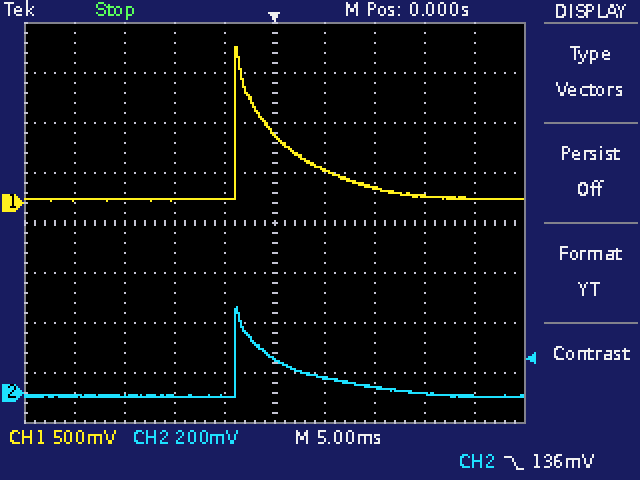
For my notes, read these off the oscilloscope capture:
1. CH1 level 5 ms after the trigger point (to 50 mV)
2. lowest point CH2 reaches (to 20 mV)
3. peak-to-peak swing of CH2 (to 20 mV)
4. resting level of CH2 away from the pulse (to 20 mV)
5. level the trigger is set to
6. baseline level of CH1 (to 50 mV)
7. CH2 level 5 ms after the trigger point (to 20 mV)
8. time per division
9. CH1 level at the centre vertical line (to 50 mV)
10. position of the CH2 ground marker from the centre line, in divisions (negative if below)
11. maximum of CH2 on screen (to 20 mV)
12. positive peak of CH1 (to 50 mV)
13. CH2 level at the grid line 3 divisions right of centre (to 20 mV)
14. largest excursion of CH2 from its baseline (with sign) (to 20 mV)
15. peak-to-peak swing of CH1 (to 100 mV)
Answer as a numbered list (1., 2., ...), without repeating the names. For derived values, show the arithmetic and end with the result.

1. 350 mV
2. -20 mV
3. 340 mV − (-20 mV) = 360 mV
4. -20 mV
5. 136 mV
6. 50 mV
7. 60 mV
8. 5 ms
9. 700 mV
10. -3.4 div
11. 340 mV
12. 1.55 V
13. 0 mV
14. 340 mV − (-20 mV) = +360 mV
15. 1.50 V
